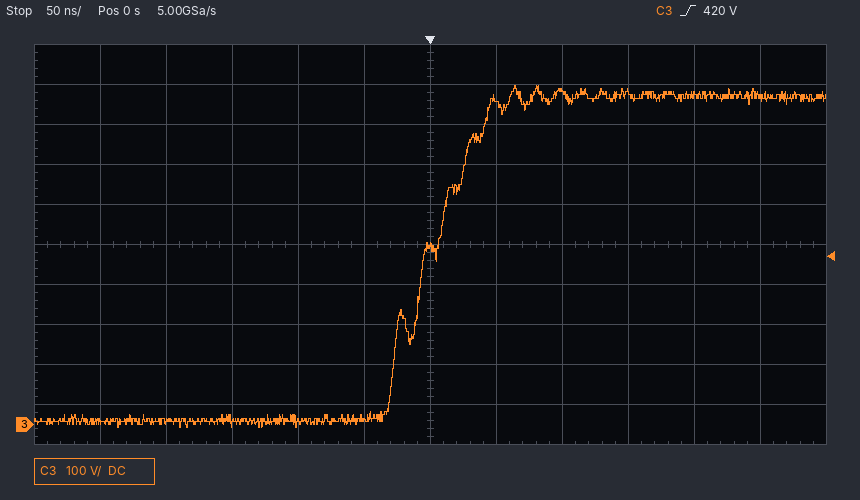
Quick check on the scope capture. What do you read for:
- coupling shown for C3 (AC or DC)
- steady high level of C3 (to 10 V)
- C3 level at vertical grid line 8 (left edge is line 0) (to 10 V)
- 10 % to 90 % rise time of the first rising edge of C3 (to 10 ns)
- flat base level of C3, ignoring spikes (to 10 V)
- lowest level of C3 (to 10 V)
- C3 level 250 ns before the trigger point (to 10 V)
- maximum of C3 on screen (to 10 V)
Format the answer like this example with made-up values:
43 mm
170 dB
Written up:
DC
820 V
830 V
70 ns
10 V
-10 V
10 V
850 V
